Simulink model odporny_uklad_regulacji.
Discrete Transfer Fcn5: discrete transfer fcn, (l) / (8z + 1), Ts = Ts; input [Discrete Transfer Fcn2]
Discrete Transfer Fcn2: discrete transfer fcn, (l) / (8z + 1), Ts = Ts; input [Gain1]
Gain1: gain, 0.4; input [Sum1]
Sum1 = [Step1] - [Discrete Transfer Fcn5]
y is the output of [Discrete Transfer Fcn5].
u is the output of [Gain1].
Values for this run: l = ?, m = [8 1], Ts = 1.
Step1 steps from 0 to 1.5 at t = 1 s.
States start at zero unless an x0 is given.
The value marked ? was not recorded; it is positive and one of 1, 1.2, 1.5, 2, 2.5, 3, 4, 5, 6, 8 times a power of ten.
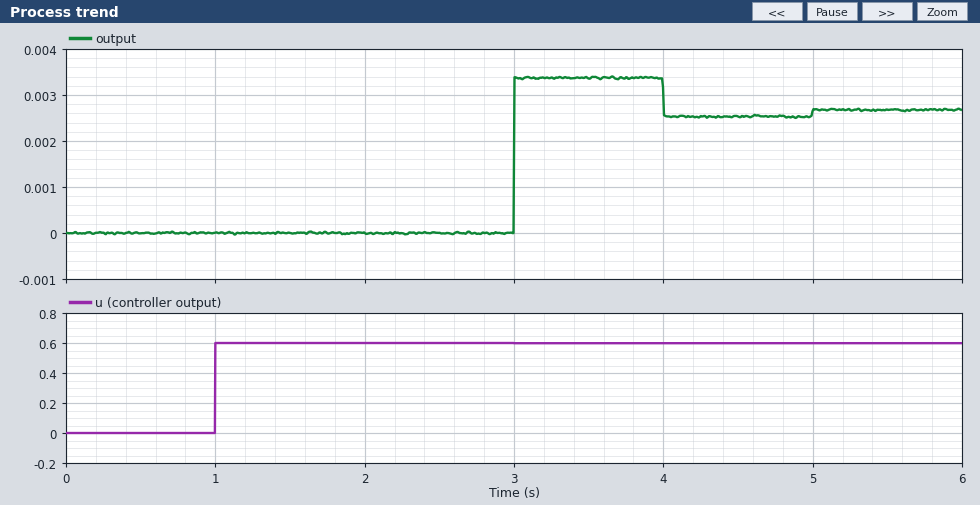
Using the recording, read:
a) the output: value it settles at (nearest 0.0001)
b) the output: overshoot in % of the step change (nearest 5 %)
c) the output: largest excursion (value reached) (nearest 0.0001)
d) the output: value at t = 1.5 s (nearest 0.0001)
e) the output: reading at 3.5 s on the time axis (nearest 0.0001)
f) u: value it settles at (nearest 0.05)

0.0027
25 %
0.0034
0.0000
0.0034
0.60
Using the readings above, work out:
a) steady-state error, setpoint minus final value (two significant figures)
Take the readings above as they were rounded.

1.5
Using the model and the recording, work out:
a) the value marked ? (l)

0.6
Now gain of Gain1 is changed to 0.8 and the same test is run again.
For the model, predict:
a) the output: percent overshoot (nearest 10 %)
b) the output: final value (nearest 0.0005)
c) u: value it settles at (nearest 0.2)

30 %
0.0055
1.2
